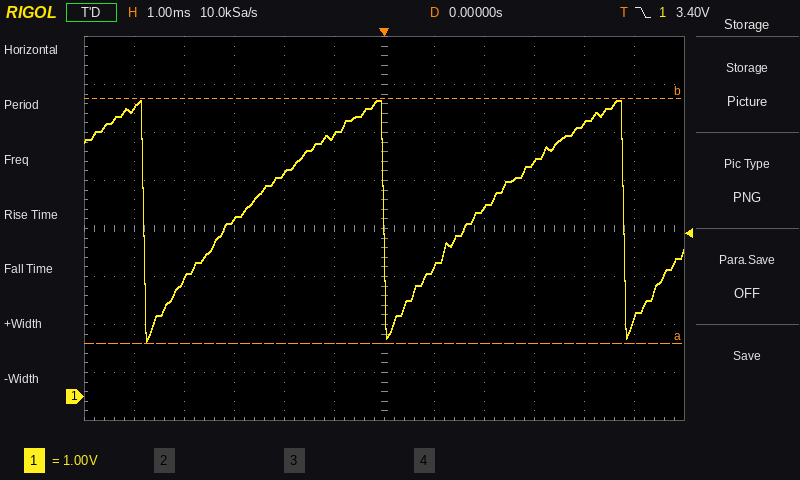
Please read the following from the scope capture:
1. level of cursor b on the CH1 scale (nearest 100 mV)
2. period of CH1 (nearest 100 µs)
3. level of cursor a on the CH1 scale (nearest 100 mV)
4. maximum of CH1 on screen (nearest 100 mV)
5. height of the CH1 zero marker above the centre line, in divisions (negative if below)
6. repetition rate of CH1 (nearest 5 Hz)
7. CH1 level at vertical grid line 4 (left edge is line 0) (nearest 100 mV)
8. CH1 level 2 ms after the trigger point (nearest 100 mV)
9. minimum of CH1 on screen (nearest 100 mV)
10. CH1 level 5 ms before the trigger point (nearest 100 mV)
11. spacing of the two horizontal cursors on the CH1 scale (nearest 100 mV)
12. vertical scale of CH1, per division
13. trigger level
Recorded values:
6.2 V
4.8 ms
1.1 V
6.2 V
-3.5 div
210 Hz
4.6 V
3.9 V
1.1 V
6.0 V
5.1 V
1 V
3.40 V
